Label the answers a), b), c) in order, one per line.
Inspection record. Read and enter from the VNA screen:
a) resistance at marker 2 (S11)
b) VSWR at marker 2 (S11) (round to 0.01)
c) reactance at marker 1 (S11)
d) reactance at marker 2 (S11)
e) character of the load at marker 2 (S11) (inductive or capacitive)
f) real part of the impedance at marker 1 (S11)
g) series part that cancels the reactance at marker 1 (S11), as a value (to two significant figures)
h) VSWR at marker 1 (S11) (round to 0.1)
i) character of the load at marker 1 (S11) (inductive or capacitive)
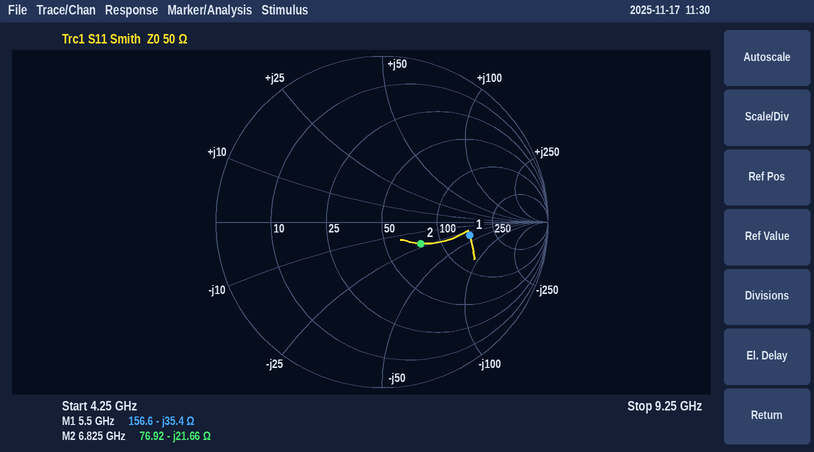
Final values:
a) 76.92 Ω
b) 1.73
c) -35.4 Ω
d) -21.66 Ω
e) capacitive
f) 156.6 Ω
g) 1.0 nH
h) 3.3
i) capacitive
